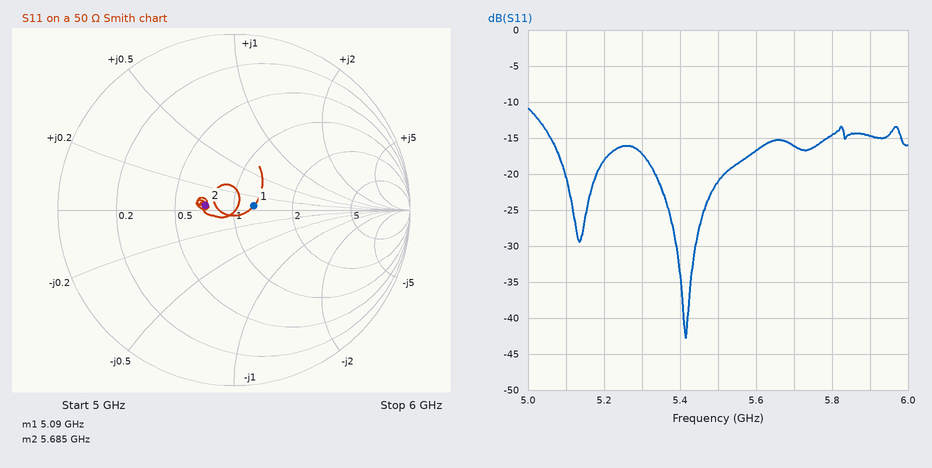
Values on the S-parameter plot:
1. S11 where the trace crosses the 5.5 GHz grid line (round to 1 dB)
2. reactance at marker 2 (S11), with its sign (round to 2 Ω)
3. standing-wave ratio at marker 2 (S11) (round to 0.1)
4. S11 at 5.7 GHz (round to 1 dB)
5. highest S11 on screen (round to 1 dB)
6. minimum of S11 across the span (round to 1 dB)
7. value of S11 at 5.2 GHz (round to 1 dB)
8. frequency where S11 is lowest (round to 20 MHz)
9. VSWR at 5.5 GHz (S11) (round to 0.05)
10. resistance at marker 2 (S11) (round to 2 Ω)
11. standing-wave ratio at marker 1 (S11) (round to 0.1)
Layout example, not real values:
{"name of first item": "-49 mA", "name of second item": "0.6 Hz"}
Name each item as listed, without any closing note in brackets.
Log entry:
{"S11 where the trace crosses the 5.5 GHz grid line": "-21 dB", "reactance at marker 2 (S11), with its sign": "+2 Ω", "standing-wave ratio at marker 2 (S11)": "1.4", "S11 at 5.7 GHz": "-16 dB", "highest S11 on screen": "-11 dB", "minimum of S11 across the span": "-43 dB", "value of S11 at 5.2 GHz": "-18 dB", "frequency where S11 is lowest": "5.42 GHz", "VSWR at 5.5 GHz (S11)": "1.20", "resistance at marker 2 (S11)": "36 Ω", "standing-wave ratio at marker 1 (S11)": "1.3"}
